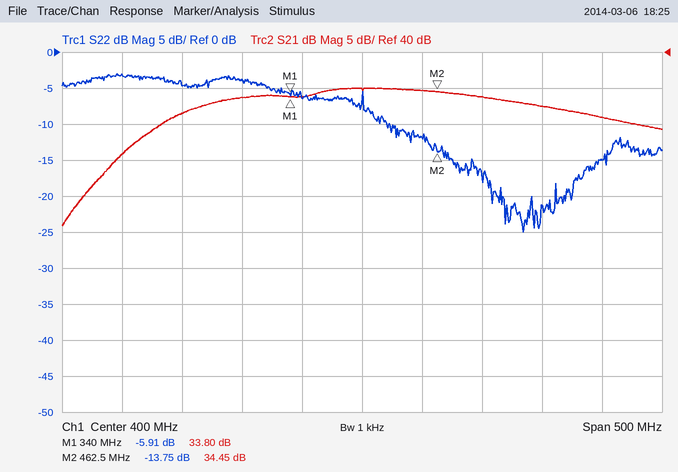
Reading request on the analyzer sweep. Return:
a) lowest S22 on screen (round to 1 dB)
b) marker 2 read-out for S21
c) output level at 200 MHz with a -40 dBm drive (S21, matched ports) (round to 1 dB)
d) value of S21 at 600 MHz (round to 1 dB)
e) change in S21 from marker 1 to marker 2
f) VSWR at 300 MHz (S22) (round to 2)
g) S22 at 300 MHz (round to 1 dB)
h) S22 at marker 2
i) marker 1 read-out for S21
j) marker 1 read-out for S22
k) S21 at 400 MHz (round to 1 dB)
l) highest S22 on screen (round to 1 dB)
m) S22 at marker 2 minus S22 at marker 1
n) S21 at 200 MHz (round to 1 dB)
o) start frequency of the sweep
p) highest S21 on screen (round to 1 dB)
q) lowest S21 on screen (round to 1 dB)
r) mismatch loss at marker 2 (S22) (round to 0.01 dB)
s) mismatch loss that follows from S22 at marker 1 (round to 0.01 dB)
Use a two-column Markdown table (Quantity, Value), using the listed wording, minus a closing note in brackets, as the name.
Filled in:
| Quantity | Value |
|---|---|
| lowest S22 on screen | -25 dB |
| marker 2 read-out for S21 | 34.45 dB |
| output level at 200 MHz with a -40 dBm drive (S21, matched ports) | -14 dBm |
| value of S21 at 600 MHz | 31 dB |
| change in S21 from marker 1 to marker 2 | 0.65 dB |
| VSWR at 300 MHz (S22) | 4 |
| S22 at 300 MHz | -4 dB |
| S22 at marker 2 | -13.75 dB |
| marker 1 read-out for S21 | 33.80 dB |
| marker 1 read-out for S22 | -5.91 dB |
| S21 at 400 MHz | 35 dB |
| highest S22 on screen | -3 dB |
| S22 at marker 2 minus S22 at marker 1 | -7.84 dB |
| S21 at 200 MHz | 26 dB |
| start frequency of the sweep | 150 MHz |
| highest S21 on screen | 35 dB |
| lowest S21 on screen | 16 dB |
| mismatch loss at marker 2 (S22) | 0.19 dB |
| mismatch loss that follows from S22 at marker 1 | 1.29 dB |
